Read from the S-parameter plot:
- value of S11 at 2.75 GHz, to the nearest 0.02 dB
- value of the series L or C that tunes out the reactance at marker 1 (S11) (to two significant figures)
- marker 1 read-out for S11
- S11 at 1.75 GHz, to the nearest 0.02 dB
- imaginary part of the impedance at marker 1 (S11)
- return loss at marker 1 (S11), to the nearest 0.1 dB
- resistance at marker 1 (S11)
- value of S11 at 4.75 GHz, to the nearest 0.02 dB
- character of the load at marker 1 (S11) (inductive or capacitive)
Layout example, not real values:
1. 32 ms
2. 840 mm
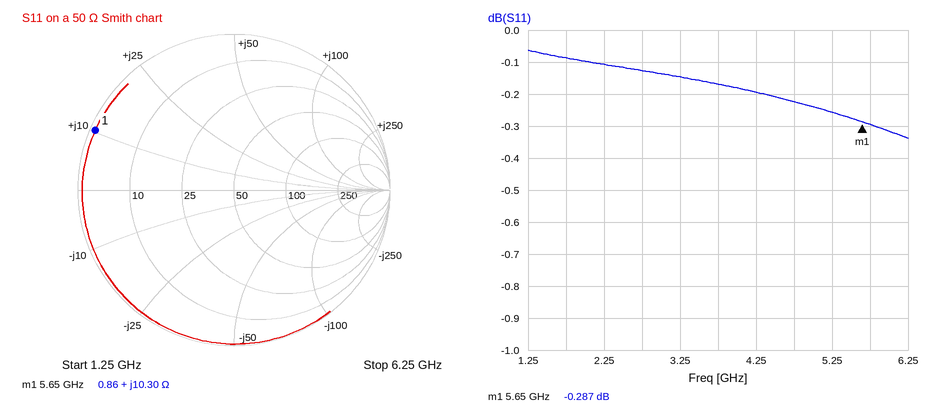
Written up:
1. -0.12 dB
2. 2.7 pF
3. -0.287 dB
4. -0.08 dB
5. +10.30 Ω
6. 0.3 dB
7. 0.86 Ω
8. -0.22 dB
9. inductive
